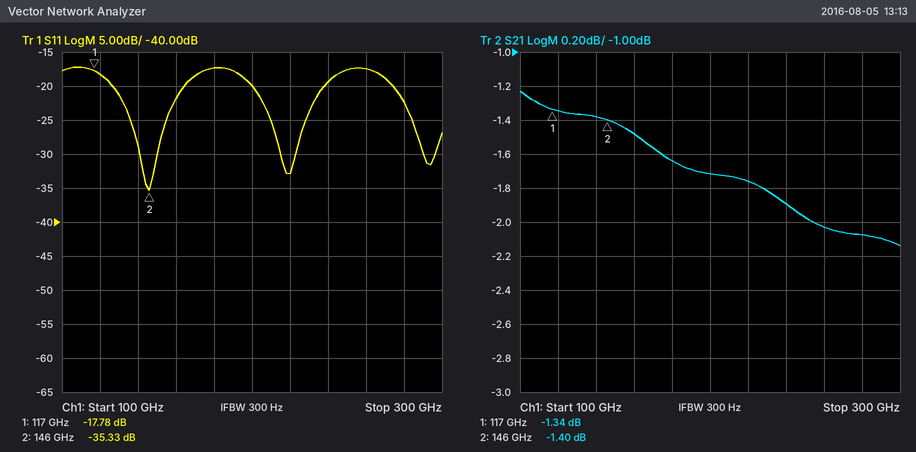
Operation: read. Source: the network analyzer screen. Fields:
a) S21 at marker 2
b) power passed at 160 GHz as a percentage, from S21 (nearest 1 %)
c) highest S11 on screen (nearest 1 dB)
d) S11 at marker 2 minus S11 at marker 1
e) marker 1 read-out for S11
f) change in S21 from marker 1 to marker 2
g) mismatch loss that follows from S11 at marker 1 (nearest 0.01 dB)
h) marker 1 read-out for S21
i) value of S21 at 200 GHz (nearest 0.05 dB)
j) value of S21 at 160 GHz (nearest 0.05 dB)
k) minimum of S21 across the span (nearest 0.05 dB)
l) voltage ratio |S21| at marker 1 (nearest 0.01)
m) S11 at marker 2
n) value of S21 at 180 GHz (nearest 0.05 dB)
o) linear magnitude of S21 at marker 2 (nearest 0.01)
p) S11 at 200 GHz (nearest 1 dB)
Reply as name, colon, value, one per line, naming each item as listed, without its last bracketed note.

S21 at marker 2: -1.40 dB
power passed at 160 GHz as a percentage, from S21: 71 %
highest S11 on screen: -17 dB
S11 at marker 2 minus S11 at marker 1: -17.55 dB
marker 1 read-out for S11: -17.78 dB
change in S21 from marker 1 to marker 2: -0.06 dB
mismatch loss that follows from S11 at marker 1: 0.07 dB
marker 1 read-out for S21: -1.34 dB
value of S21 at 200 GHz: -1.70 dB
value of S21 at 160 GHz: -1.50 dB
minimum of S21 across the span: -2.15 dB
voltage ratio |S21| at marker 1: 0.86
S11 at marker 2: -35.33 dB
value of S21 at 180 GHz: -1.65 dB
linear magnitude of S21 at marker 2: 0.85
S11 at 200 GHz: -20 dB
